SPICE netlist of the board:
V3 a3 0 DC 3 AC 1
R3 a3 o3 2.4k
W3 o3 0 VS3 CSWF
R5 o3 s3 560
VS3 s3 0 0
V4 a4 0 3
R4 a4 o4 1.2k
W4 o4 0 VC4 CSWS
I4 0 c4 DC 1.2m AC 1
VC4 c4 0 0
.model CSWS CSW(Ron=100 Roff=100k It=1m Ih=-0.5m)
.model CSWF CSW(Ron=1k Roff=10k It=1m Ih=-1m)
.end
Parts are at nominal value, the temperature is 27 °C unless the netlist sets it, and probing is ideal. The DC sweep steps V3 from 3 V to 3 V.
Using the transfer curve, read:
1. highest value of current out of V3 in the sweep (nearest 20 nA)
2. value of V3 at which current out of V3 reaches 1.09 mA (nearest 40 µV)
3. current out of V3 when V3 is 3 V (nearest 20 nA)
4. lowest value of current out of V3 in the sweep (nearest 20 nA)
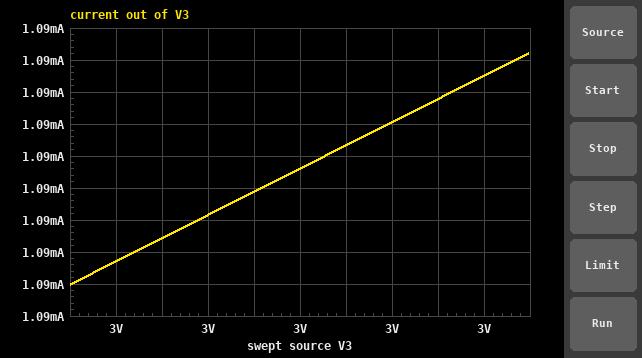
1.08772 mA
2.99956 V
1.08722 mA
1.08700 mA
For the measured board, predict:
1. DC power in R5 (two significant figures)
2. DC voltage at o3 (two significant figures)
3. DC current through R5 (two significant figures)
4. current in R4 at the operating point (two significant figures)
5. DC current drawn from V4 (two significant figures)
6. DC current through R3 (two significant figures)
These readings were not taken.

270 µW
390 mV
700 µA
2.3 mA
2.3 mA
1.1 mA
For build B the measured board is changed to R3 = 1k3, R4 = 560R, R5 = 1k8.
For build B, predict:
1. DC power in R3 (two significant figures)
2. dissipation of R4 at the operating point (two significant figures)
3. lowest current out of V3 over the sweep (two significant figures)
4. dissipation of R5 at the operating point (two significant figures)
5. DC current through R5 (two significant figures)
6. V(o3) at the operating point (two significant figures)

3.1 mW
12 mW
1.5 mA
550 µW
550 µA
990 mV
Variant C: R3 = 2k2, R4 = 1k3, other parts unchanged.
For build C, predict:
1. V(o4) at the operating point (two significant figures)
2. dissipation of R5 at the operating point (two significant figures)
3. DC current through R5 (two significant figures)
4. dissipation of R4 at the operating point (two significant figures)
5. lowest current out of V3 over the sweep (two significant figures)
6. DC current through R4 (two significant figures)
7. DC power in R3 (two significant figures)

210 mV
320 µW
750 µA
6.0 mW
1.2 mA
2.1 mA
3.0 mW
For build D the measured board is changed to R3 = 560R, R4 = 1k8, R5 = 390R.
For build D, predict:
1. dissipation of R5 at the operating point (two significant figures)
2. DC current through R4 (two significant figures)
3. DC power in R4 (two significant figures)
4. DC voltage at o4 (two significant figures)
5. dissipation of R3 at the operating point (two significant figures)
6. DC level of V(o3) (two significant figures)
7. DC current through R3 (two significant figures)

2.6 mW
1.6 mA
4.5 mW
160 mV
7.1 mW
1.0 V
3.6 mA
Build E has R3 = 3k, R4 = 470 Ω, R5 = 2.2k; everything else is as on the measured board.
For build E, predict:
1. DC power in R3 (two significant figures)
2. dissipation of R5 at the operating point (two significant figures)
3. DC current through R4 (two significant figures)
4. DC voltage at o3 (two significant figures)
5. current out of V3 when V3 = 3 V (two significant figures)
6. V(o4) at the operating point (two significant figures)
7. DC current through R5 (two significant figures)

2.0 mW
140 µW
5.3 mA
560 mV
810 µA
530 mV
250 µA
